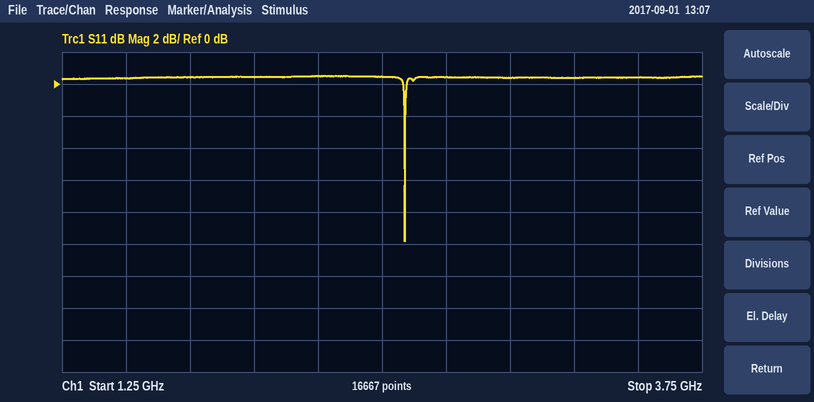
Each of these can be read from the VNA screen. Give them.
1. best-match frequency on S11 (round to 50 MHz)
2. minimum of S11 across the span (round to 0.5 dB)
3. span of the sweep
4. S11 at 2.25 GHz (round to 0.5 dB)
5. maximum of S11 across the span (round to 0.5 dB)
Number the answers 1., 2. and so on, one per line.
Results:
1. 2.60 GHz
2. -10.0 dB
3. 2.5 GHz
4. 0.5 dB
5. 0.5 dB
